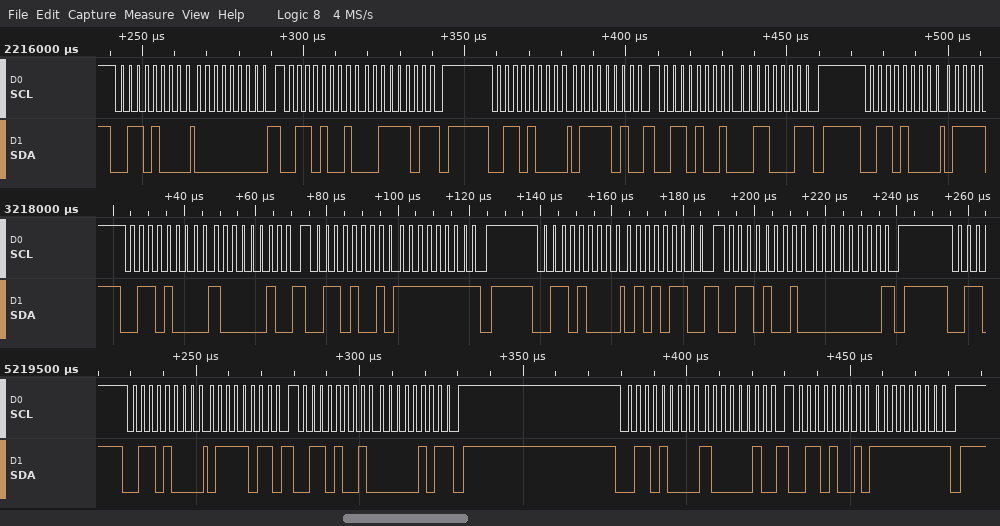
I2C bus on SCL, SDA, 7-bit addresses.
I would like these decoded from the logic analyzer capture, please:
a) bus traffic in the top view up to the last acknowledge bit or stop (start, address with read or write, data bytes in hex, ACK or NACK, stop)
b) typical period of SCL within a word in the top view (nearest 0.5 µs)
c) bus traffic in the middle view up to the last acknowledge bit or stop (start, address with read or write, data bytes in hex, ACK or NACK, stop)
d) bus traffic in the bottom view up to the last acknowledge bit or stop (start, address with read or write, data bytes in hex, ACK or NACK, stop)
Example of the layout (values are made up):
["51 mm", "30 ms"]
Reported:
["start, address 34 write ACK, 00 ACK, repeated start, address 34 read ACK, 3D NACK, stop, start, address 34 write ACK, 7A ACK, repeated start, address 34 read ACK, 31 NACK, stop, start, address 34 write ACK", "2.5 µs", "start, address 34 write ACK, 82 ACK, repeated start, address 34 read ACK, FF NACK, stop, start, address 34 write ACK, 56 ACK, repeated start, address 34 read ACK, 00 NACK, stop", "start, address 34 write ACK, 7B ACK, repeated start, address 34 read ACK, 05 NACK, stop, start, address 34 write ACK, 82 ACK, repeated start, address 34 read ACK, FF NACK, stop"]
